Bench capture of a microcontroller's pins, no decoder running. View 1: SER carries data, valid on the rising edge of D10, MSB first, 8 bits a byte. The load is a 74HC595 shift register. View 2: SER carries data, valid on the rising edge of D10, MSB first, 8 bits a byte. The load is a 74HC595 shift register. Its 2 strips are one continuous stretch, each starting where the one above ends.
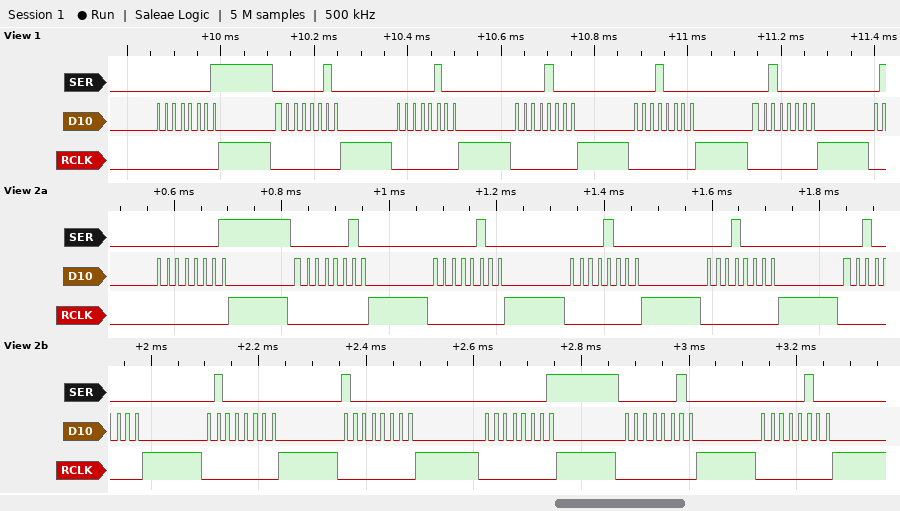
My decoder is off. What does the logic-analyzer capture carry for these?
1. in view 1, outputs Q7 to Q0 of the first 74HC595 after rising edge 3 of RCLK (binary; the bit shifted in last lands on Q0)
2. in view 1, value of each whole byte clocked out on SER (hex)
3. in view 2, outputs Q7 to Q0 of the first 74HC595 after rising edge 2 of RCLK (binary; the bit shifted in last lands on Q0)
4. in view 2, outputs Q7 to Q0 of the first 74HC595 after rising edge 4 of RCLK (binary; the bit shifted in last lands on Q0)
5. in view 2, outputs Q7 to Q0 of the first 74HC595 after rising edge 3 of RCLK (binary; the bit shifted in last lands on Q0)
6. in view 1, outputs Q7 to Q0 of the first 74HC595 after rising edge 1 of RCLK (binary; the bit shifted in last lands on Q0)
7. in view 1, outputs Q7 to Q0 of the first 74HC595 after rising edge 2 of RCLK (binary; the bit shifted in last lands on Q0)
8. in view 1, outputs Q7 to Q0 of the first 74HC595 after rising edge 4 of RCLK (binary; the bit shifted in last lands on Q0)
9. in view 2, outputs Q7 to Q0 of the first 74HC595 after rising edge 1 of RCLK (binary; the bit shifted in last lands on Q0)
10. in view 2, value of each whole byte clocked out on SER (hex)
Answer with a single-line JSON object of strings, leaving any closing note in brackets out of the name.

{"in view 1, outputs Q7 to Q0 of the first 74HC595 after rising edge 3 of RCLK": "00000100", "in view 1, value of each whole byte clocked out on SER": "01 02 04 08 10 20", "in view 2, outputs Q7 to Q0 of the first 74HC595 after rising edge 2 of RCLK": "00000010", "in view 2, outputs Q7 to Q0 of the first 74HC595 after rising edge 4 of RCLK": "00001000", "in view 2, outputs Q7 to Q0 of the first 74HC595 after rising edge 3 of RCLK": "00000100", "in view 1, outputs Q7 to Q0 of the first 74HC595 after rising edge 1 of RCLK": "00000001", "in view 1, outputs Q7 to Q0 of the first 74HC595 after rising edge 2 of RCLK": "00000010", "in view 1, outputs Q7 to Q0 of the first 74HC595 after rising edge 4 of RCLK": "00001000", "in view 2, outputs Q7 to Q0 of the first 74HC595 after rising edge 1 of RCLK": "00000001", "in view 2, value of each whole byte clocked out on SER": "01 02 04 08 10 20 40 80 01 02 04"}
